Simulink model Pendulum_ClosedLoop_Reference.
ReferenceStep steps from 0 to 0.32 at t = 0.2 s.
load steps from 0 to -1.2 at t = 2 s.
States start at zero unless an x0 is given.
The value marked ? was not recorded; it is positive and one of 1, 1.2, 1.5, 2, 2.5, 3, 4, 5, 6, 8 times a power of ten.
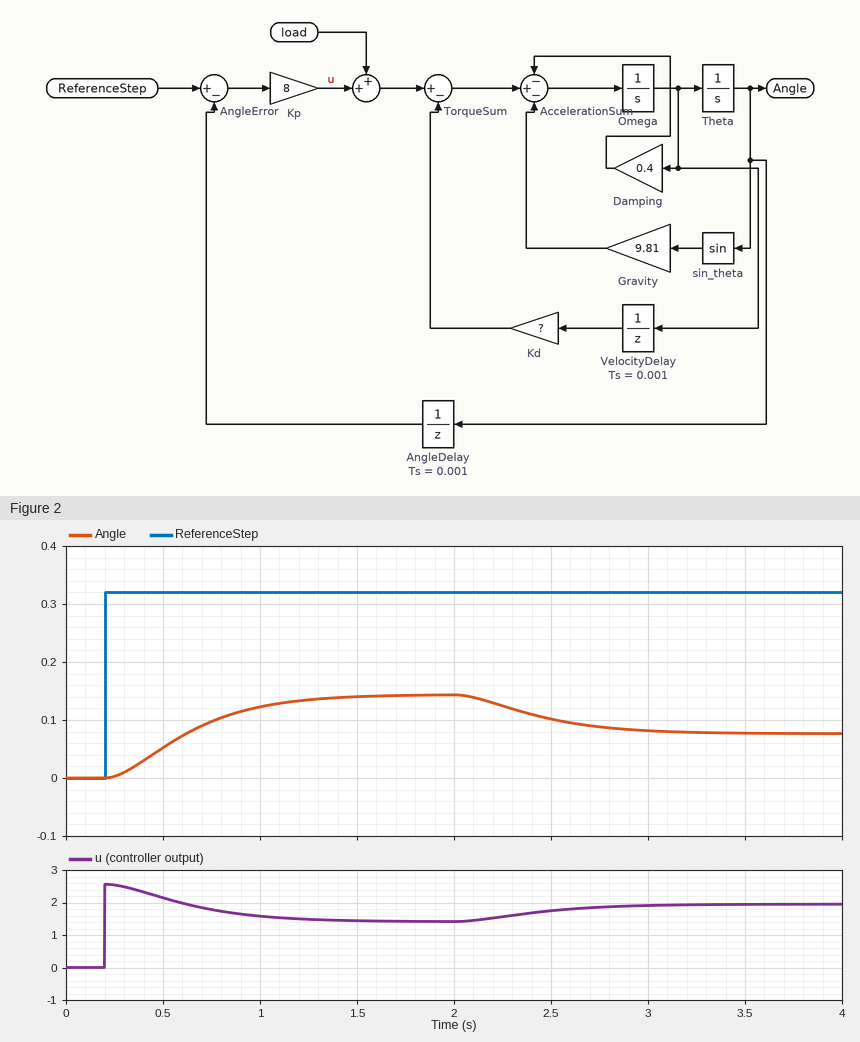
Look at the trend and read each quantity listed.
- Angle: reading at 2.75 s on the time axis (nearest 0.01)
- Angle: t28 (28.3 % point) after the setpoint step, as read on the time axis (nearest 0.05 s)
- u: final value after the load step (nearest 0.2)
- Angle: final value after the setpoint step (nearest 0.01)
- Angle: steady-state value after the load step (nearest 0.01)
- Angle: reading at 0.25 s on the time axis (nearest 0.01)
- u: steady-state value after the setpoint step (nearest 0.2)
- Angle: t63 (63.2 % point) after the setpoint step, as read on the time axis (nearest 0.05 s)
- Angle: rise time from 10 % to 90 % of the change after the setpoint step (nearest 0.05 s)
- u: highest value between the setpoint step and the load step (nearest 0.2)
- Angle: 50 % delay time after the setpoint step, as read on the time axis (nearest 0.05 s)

0.09
0.45 s
2.0
0.14
0.08
0.00
1.4
0.70 s
0.80 s
2.6
0.60 s
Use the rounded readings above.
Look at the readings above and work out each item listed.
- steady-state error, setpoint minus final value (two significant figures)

0.18
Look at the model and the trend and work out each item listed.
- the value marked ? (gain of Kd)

8
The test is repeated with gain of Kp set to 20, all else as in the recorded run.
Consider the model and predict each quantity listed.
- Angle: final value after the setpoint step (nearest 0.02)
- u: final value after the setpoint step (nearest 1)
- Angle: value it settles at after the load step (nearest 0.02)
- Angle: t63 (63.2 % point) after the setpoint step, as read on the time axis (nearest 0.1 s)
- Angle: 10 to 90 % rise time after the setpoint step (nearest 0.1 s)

0.22
2
0.18
0.5 s
0.4 s
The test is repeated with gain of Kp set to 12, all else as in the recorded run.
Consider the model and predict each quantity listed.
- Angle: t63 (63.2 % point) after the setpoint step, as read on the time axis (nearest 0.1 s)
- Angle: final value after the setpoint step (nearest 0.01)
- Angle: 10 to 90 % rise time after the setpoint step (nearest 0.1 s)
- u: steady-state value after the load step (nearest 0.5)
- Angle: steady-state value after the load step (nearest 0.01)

0.6 s
0.18
0.6 s
2.5
0.12
